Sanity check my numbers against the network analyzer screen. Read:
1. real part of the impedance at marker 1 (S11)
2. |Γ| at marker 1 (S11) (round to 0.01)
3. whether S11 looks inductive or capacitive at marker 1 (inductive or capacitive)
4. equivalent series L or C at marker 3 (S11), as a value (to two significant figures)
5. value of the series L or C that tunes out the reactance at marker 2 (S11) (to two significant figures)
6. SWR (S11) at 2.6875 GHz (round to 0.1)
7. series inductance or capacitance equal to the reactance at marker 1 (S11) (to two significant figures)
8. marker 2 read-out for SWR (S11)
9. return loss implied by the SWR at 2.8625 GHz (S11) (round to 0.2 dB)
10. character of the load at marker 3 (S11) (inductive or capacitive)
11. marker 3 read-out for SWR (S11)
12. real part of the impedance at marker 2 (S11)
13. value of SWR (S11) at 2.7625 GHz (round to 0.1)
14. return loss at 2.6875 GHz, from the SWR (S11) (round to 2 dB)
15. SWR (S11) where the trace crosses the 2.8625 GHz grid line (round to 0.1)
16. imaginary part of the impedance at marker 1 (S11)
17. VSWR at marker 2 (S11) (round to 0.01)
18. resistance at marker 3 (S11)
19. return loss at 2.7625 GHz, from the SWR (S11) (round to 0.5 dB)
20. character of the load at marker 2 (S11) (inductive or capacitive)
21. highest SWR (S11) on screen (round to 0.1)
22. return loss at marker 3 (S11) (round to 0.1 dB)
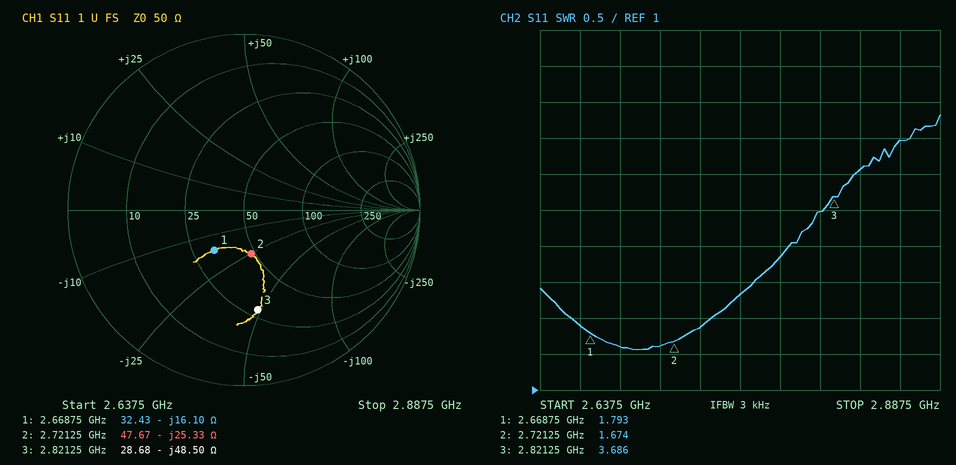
32.43 Ω
0.28
capacitive
1.2 pF
1.5 nH
1.6
3.7 pF
1.674
4.0 dB
capacitive
3.686
47.67 Ω
2.3
12 dB
4.5
-16.10 Ω
1.67
28.68 Ω
8.0 dB
capacitive
4.8
4.8 dB
